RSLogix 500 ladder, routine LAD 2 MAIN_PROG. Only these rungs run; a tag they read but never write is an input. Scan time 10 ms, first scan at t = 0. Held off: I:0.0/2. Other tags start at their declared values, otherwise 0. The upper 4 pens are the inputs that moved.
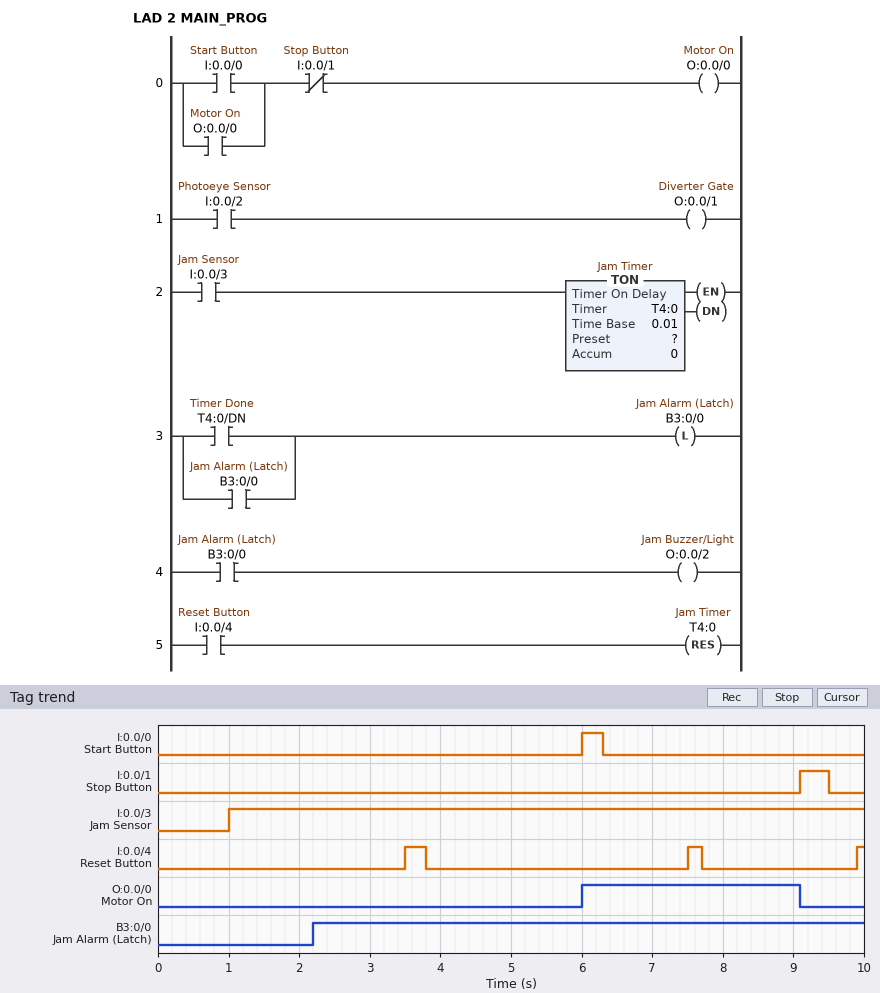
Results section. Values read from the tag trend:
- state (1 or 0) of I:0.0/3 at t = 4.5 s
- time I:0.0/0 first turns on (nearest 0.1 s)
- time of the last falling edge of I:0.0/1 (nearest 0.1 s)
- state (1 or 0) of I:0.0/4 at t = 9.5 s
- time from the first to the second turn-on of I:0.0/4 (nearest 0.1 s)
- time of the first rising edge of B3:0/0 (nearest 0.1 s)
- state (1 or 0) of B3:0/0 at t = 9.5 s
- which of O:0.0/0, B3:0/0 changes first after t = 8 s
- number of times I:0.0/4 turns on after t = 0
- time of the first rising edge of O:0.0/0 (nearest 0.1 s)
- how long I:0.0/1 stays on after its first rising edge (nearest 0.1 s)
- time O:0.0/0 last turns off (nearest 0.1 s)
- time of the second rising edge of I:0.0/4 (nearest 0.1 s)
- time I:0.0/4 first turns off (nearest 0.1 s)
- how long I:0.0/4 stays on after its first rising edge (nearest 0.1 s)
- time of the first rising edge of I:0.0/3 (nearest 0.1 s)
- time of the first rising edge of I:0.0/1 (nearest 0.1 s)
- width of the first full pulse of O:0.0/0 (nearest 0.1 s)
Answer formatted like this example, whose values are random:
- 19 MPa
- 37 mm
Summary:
- 1
- 6.0 s
- 9.5 s
- 0
- 4.0 s
- 2.2 s
- 1
- O:0.0/0
- 3
- 6.0 s
- 0.4 s
- 9.1 s
- 7.5 s
- 3.8 s
- 0.3 s
- 1.0 s
- 9.1 s
- 3.1 s
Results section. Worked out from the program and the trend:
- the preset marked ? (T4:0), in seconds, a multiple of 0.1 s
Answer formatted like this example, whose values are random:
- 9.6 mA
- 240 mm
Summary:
- 1.2 s
